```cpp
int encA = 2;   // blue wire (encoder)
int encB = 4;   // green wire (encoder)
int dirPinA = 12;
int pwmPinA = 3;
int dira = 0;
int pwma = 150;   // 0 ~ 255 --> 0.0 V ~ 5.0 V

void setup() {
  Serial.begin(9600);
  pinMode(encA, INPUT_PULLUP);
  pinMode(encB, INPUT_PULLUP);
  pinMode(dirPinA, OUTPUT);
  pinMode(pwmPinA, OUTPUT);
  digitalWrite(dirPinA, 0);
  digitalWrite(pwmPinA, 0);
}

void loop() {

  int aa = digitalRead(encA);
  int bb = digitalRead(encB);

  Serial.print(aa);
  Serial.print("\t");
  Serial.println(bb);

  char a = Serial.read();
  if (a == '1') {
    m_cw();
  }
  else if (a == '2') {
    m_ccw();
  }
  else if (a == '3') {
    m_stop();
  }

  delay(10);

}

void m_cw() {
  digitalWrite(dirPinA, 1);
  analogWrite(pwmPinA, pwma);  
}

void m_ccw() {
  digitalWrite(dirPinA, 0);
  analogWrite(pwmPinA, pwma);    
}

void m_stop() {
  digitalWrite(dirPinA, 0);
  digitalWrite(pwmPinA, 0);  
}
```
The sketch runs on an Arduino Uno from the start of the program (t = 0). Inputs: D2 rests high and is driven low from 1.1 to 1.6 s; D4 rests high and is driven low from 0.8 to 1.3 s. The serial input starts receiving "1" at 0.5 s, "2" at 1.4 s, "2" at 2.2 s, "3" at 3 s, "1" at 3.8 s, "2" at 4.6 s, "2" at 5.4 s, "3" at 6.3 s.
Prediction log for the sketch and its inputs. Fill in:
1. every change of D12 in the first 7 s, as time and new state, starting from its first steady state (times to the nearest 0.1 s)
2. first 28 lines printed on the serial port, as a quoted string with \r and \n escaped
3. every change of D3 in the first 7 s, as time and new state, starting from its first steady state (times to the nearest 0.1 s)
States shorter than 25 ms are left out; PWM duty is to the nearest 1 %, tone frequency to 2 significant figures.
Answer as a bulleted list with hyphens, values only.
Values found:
- 0 s low; 0.5 s high; 1.4 s low; 3.8 s high; 4.6 s low
- "1\t1\r\n1\t1\r\n1\t1\r\n1\t1\r\n1\t1\r\n1\t1\r\n1\t1\r\n1\t1\r\n1\t1\r\n1\t1\r\n1\t1\r\n1\t1\r\n1\t1\r\n1\t1\r\n1\t1\r\n1\t1\r\n1\t1\r\n1\t1\r\n1\t1\r\n1\t1\r\n1\t1\r\n1\t1\r\n1\t1\r\n1\t1\r\n1\t1\r\n1\t1\r\n1\t1\r\n1\t1\r\n"
- 0 s low; 0.5 s PWM 59 %; 3 s low; 3.8 s PWM 59 %; 6.3 s low
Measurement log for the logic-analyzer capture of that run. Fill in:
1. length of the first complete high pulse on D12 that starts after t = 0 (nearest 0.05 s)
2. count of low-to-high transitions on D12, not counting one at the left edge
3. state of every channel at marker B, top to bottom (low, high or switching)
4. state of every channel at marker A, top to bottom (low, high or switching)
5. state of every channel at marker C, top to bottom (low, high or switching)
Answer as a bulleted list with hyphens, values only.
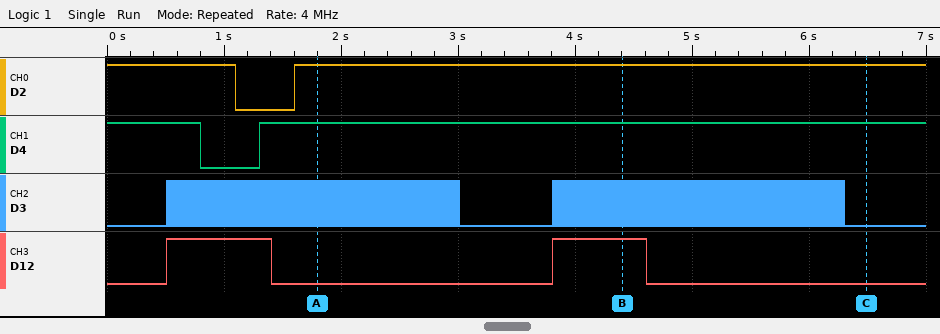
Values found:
- 0.90 s
- 2
- D2 high, D4 high, D3 switching, D12 high
- D2 high, D4 high, D3 switching, D12 low
- D2 high, D4 high, D3 low, D12 low
